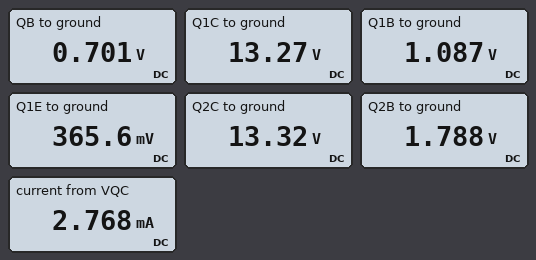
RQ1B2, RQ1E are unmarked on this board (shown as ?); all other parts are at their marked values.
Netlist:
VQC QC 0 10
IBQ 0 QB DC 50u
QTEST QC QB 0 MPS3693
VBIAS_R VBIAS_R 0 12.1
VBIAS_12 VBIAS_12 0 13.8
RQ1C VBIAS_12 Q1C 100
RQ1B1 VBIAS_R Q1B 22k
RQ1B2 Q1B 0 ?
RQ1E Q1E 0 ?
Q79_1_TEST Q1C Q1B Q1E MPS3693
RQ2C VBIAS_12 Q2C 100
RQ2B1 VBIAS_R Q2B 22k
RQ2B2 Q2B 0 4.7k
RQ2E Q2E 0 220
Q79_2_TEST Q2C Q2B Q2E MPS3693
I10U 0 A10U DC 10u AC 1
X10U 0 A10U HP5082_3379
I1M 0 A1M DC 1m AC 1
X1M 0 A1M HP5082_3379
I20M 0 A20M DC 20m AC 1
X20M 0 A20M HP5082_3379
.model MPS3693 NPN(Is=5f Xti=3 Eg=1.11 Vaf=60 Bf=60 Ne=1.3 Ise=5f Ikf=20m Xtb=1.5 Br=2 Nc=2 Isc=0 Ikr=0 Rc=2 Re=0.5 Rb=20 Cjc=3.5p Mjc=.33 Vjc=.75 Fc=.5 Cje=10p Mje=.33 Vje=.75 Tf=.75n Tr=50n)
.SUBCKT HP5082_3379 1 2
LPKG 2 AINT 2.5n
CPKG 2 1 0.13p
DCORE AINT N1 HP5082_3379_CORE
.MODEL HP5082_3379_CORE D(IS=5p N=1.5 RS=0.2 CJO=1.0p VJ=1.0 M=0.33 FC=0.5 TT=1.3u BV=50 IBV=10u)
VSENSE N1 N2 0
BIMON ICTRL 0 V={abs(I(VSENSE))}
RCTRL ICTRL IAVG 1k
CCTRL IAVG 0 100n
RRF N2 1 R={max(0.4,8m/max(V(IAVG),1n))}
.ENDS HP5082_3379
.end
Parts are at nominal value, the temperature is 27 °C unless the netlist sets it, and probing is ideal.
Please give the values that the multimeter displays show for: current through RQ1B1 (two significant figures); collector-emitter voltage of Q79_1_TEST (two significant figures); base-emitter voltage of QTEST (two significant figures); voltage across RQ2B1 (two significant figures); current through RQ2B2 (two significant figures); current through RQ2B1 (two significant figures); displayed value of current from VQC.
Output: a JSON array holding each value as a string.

["500 µA", "13 V", "700 mV", "10 V", "380 µA", "470 µA", "2.768 mA"]
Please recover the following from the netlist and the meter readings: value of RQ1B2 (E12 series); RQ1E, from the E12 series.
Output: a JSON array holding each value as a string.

["2.7 kΩ", "68 Ω"]
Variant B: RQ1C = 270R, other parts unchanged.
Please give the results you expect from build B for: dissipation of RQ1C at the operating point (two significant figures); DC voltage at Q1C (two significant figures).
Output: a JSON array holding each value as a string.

["7.4 mW", "12 V"]
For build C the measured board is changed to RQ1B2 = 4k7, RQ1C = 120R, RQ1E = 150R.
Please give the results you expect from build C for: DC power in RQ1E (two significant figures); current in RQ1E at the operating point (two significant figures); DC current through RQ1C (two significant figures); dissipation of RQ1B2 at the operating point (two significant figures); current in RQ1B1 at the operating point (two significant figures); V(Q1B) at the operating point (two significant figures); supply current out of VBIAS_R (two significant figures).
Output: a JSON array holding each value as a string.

["5.9 mW", "6.3 mA", "6.2 mA", "590 µW", "470 µA", "1.7 V", "940 µA"]
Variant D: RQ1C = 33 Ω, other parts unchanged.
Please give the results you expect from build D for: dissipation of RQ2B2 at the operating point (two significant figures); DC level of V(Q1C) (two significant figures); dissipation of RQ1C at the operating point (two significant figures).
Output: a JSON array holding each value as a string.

["680 µW", "14 V", "920 µW"]
